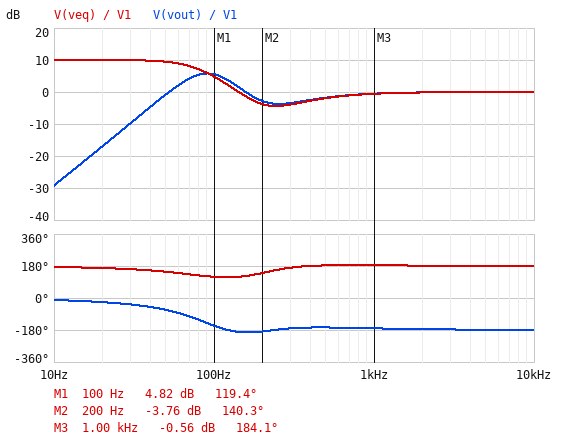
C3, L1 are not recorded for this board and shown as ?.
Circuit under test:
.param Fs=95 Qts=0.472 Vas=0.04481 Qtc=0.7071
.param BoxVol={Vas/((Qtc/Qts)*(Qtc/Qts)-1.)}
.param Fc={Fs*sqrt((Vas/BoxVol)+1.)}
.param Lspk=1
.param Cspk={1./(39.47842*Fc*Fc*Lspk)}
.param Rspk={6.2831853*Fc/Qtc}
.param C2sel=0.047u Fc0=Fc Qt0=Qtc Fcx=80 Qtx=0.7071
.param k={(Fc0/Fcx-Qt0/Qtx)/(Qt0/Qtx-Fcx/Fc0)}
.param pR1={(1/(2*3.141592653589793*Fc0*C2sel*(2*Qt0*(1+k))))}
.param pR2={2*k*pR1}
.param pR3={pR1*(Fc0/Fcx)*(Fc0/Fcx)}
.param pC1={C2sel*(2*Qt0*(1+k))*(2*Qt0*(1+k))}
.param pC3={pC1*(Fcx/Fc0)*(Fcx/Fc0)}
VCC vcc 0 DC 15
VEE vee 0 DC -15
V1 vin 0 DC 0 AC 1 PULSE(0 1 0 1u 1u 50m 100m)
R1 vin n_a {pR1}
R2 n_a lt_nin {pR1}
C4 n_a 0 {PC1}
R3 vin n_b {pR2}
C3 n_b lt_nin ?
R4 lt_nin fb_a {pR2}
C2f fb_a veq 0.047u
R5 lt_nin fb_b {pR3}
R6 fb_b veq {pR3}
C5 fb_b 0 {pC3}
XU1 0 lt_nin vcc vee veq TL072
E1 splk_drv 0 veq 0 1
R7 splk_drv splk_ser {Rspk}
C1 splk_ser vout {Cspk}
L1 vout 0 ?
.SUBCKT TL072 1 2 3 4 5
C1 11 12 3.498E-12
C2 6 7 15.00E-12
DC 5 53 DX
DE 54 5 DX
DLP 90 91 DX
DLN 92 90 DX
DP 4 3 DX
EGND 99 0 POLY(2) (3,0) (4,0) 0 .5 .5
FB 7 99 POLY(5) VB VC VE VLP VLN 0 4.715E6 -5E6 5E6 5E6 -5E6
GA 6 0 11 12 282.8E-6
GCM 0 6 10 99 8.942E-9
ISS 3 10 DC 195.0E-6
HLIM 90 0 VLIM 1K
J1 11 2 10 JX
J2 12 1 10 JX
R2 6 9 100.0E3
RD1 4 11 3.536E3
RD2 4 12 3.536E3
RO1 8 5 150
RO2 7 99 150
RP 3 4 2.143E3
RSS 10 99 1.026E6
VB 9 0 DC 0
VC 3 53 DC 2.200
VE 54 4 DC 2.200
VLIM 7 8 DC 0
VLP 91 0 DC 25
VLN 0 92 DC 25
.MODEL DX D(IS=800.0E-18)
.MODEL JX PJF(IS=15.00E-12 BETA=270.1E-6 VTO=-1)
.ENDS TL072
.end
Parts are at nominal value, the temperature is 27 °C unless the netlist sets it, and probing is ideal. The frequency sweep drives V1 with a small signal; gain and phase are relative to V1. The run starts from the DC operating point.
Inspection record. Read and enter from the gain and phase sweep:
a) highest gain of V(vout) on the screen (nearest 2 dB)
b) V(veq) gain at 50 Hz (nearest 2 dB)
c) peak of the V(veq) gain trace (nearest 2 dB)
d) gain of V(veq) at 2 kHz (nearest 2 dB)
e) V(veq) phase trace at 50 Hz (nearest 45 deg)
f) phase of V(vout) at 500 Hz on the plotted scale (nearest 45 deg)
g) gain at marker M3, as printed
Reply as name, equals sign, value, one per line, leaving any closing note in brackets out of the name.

highest gain of V(vout) on the screen = 6 dB
V(veq) gain at 50 Hz = 10 dB
peak of the V(veq) gain trace = 10 dB
gain of V(veq) at 2 kHz = 0 dB
V(veq) phase trace at 50 Hz = 135 deg
phase of V(vout) at 500 Hz on the plotted scale = -180 deg
gain at marker M3, as printed = -0.56 dB
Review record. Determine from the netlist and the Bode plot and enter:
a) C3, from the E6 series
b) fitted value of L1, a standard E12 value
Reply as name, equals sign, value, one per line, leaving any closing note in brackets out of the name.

C3, from the E6 series = 22 nF
fitted value of L1, a standard E12 value = 2.2 H
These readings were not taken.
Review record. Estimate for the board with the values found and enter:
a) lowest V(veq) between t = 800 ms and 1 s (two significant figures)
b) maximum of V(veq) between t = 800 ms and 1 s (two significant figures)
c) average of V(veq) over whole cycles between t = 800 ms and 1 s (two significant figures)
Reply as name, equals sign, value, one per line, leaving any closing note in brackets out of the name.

lowest V(veq) between t = 800 ms and 1 s = -3.3 V
maximum of V(veq) between t = 800 ms and 1 s = 140 mV
average of V(veq) over whole cycles between t = 800 ms and 1 s = -1.6 V
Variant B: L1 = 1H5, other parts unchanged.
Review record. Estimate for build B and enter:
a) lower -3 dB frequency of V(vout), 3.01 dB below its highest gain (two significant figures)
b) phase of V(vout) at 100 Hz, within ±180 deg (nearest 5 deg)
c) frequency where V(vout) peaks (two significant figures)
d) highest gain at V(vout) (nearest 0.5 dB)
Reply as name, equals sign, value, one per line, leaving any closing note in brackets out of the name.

lower -3 dB frequency of V(vout), 3.01 dB below its highest gain = 65 Hz
phase of V(vout) at 100 Hz, within ±180 deg = -135 deg
frequency where V(vout) peaks = 100 Hz
highest gain at V(vout) = 2.0 dB
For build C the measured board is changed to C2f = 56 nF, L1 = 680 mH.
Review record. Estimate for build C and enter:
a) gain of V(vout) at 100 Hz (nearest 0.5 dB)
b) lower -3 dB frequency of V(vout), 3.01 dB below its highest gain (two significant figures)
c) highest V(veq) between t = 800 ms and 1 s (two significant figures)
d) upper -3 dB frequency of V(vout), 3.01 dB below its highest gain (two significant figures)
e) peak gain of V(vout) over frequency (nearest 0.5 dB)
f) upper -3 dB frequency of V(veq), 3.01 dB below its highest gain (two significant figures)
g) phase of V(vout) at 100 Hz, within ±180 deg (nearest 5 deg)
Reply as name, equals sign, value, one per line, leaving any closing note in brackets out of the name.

gain of V(vout) at 100 Hz = -7.5 dB
lower -3 dB frequency of V(vout), 3.01 dB below its highest gain = 460 Hz
highest V(veq) between t = 800 ms and 1 s = 80 mV
upper -3 dB frequency of V(vout), 3.01 dB below its highest gain = 550 kHz
peak gain of V(vout) over frequency = 0 dB
upper -3 dB frequency of V(veq), 3.01 dB below its highest gain = 70 Hz
phase of V(vout) at 100 Hz, within ±180 deg = -115 deg
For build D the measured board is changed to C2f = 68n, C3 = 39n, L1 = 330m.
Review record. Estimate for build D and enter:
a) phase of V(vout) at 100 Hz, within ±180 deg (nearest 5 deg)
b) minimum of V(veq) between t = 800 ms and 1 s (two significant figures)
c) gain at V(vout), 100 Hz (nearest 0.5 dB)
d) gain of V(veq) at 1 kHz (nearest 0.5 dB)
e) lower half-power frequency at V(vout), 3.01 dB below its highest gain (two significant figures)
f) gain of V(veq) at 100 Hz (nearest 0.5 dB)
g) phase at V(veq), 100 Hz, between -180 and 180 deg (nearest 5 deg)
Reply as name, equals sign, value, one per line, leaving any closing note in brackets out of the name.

phase of V(vout) at 100 Hz, within ±180 deg = -95 deg
minimum of V(veq) between t = 800 ms and 1 s = -3.2 V
gain at V(vout), 100 Hz = -15.5 dB
gain of V(veq) at 1 kHz = 0 dB
lower half-power frequency at V(vout), 3.01 dB below its highest gain = 570 Hz
gain of V(veq) at 100 Hz = 2.5 dB
phase at V(veq), 100 Hz, between -180 and 180 deg = 135 deg
